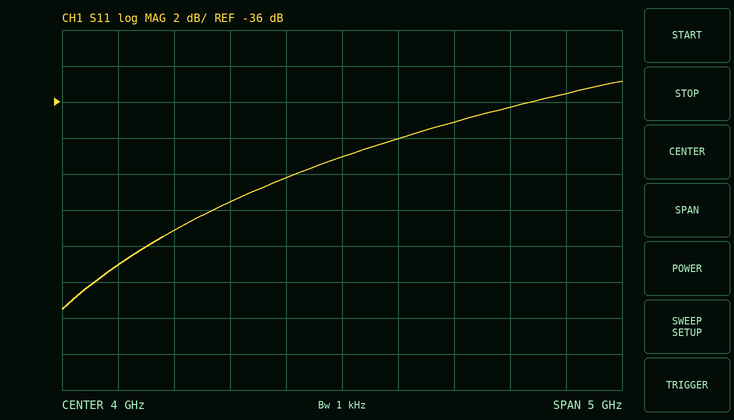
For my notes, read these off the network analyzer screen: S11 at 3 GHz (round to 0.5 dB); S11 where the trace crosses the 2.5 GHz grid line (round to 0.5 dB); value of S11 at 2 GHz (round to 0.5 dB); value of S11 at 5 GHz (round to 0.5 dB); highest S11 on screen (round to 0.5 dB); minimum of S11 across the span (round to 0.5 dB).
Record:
-41.5 dB
-43.0 dB
-45.0 dB
-37.0 dB
-35.0 dB
-47.5 dB
